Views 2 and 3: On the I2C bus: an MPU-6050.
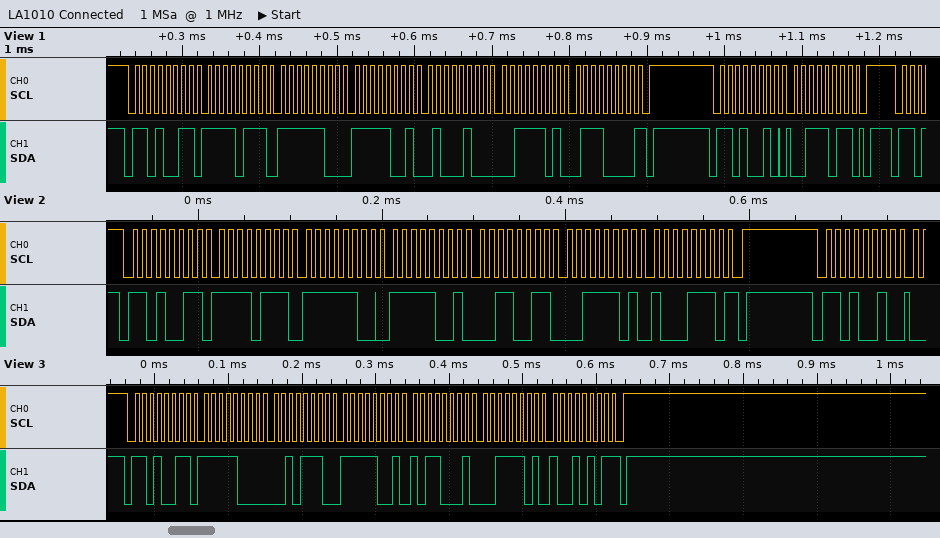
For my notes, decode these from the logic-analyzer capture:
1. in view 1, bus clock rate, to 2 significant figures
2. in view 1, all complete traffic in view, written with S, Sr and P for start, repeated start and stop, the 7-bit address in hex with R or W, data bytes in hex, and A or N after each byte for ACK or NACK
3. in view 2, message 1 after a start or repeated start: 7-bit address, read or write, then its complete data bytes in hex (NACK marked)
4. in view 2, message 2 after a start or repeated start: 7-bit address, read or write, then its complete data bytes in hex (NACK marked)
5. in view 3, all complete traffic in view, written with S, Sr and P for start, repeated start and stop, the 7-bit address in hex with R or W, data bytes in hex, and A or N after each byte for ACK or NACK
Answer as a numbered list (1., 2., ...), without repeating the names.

1. 100 kHz
2. S 69R A F7 A FC A F9 A 44 A 3D A 70 N P S 69W A 3B A P
3. 0x69 read: F7 FC F9 33 3D 8E NACK
4. 0x69 write
5. S 69R A F8 A 2E A F9 A B1 A 3D A 95 N P
